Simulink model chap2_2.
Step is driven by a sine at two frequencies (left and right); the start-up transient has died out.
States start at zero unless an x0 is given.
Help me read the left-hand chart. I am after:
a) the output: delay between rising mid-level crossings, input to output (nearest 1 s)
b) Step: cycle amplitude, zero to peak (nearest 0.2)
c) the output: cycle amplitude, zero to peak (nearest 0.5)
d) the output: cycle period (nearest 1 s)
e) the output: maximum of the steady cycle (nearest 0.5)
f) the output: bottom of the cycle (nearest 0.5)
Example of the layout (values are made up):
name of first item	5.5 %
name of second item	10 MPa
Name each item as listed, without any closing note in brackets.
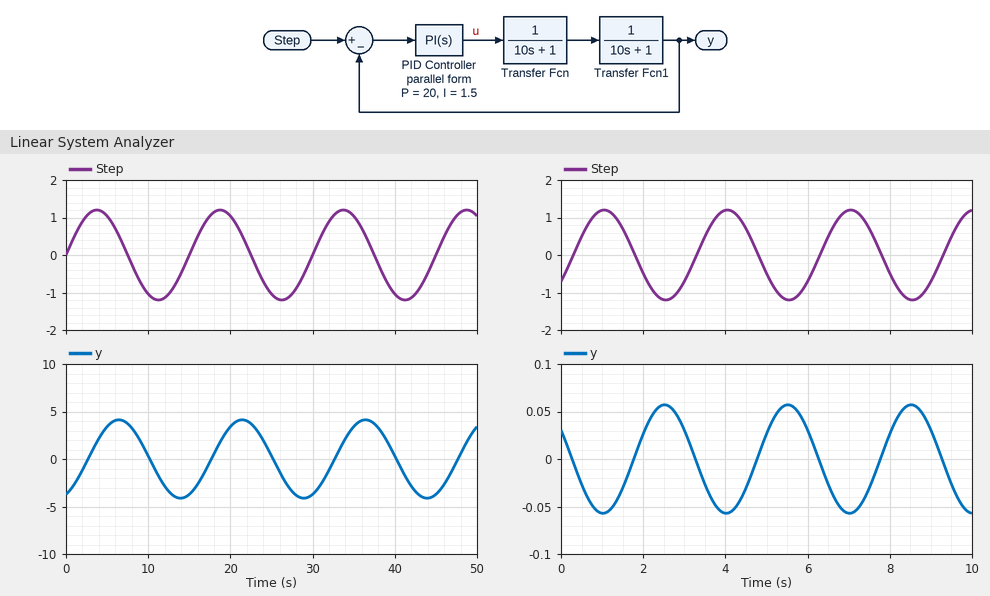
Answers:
the output: delay between rising mid-level crossings, input to output	3 s
Step: cycle amplitude, zero to peak	1.2
the output: cycle amplitude, zero to peak	4.0
the output: cycle period	15 s
the output: maximum of the steady cycle	4.0
the output: bottom of the cycle	-4.0
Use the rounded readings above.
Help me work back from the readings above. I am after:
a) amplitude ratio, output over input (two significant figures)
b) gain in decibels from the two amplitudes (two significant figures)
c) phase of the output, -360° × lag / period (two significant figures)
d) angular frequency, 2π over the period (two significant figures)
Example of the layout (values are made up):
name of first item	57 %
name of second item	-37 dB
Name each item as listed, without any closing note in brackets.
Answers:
amplitude ratio, output over input	3.3
gain in decibels from the two amplitudes	10 dB
phase of the output, -360° × lag / period	-72°
angular frequency, 2π over the period	0.42 rad/s
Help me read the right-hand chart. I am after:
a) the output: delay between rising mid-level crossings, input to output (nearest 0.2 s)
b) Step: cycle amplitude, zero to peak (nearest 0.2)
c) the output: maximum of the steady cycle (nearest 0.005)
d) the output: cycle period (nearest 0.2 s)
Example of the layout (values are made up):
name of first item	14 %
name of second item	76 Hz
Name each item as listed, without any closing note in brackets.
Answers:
the output: delay between rising mid-level crossings, input to output	1.4 s
Step: cycle amplitude, zero to peak	1.2
the output: maximum of the steady cycle	0.055
the output: cycle period	3.0 s
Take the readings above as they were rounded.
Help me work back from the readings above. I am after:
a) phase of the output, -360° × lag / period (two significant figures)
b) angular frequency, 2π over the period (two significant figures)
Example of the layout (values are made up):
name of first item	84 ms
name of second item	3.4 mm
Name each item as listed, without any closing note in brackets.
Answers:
phase of the output, -360° × lag / period	-170°
angular frequency, 2π over the period	2.1 rad/s
